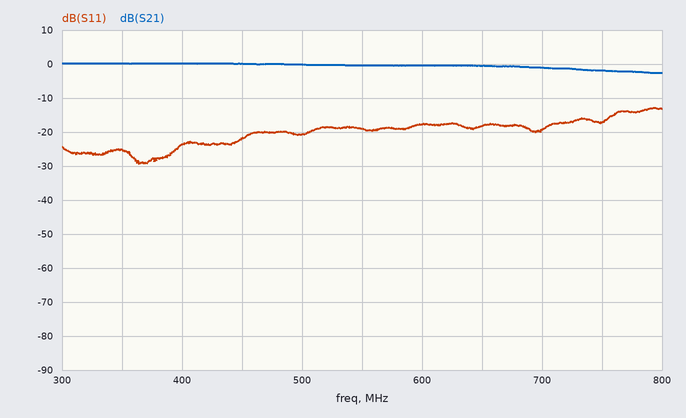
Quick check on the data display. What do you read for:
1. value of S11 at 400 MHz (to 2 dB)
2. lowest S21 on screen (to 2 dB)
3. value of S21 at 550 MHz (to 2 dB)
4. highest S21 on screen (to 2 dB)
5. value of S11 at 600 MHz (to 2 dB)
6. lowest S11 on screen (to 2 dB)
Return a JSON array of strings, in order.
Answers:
["-24 dB", "-2 dB", "0 dB", "0 dB", "-18 dB", "-30 dB"]
